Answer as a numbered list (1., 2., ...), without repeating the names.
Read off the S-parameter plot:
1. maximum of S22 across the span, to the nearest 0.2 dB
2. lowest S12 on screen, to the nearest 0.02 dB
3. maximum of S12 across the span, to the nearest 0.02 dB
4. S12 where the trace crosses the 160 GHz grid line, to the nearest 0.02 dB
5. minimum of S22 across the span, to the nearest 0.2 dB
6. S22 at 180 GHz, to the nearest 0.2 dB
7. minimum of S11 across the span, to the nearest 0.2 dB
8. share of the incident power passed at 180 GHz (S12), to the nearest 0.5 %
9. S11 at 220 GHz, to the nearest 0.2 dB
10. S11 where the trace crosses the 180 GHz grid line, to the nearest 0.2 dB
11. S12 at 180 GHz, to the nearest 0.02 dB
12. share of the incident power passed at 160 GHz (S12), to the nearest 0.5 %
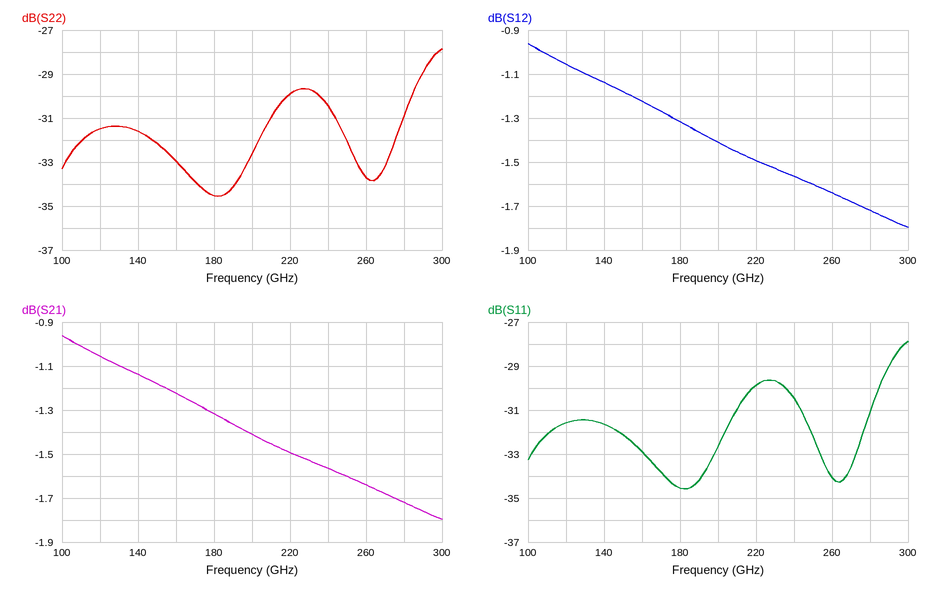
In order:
1. -27.8 dB
2. -1.80 dB
3. -0.96 dB
4. -1.22 dB
5. -34.6 dB
6. -34.6 dB
7. -34.6 dB
8. 74.0 %
9. -29.8 dB
10. -34.6 dB
11. -1.32 dB
12. 75.5 %
